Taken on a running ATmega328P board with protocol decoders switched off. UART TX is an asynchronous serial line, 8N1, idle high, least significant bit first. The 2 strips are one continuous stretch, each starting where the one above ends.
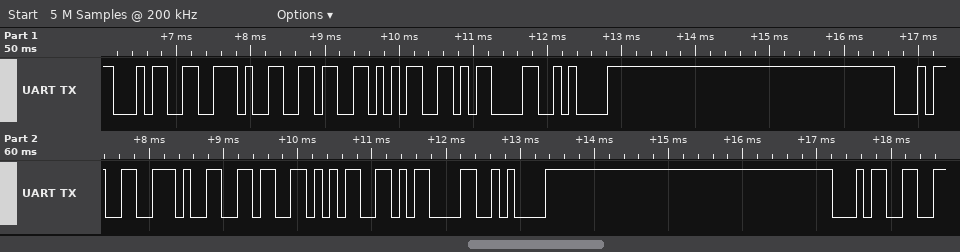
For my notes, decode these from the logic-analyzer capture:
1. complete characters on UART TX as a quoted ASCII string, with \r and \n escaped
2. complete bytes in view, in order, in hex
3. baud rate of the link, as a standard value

"4.65\r\n4.65\r\n4"
0x34 0x2E 0x36 0x35 0x0D 0x0A 0x34 0x2E 0x36 0x35 0x0D 0x0A 0x34
9600 baud
